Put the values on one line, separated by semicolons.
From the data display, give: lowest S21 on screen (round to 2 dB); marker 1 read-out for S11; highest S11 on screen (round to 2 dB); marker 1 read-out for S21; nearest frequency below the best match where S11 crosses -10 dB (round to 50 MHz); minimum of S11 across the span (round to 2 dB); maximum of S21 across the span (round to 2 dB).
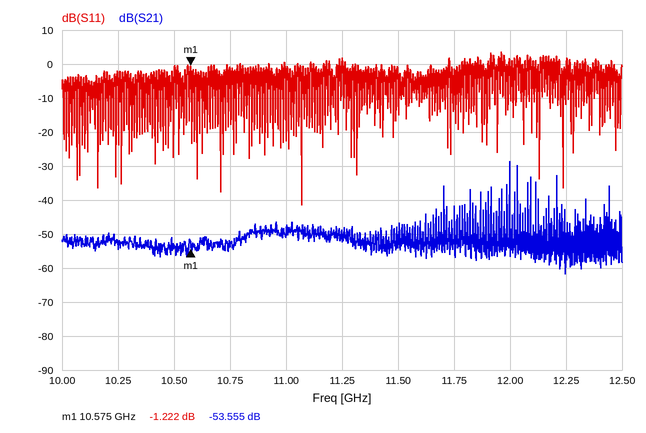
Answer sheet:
-62 dB; -1.222 dB; 4 dB; -53.555 dB; 11.05 GHz; -42 dB; -28 dB
